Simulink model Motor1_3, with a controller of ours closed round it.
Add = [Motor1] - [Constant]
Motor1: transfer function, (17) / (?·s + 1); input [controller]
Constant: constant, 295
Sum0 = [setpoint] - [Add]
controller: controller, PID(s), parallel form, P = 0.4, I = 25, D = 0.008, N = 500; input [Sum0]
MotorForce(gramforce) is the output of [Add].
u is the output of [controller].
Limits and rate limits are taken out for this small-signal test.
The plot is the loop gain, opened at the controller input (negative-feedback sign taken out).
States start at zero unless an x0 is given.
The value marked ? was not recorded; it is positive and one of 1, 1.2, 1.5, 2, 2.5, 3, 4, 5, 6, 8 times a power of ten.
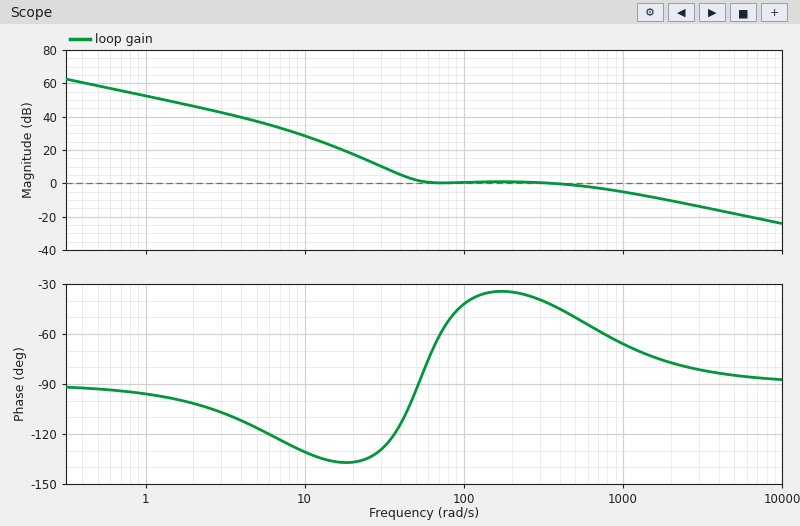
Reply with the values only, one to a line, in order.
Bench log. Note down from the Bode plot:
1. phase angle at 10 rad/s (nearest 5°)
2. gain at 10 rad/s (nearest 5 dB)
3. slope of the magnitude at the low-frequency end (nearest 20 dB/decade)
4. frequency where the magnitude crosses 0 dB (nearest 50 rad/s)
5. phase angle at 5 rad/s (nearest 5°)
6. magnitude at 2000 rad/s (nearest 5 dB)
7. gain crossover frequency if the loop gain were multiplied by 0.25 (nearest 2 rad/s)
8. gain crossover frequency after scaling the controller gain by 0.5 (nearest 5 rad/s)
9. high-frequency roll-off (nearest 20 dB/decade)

-130°
30 dB
-20 dB/decade
350 rad/s
-115°
-10 dB
28 rad/s
40 rad/s
-20 dB/decade
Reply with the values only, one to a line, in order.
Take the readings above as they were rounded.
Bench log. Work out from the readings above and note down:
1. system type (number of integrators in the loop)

1
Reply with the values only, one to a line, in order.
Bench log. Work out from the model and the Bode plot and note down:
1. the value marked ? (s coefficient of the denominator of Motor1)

0.12
